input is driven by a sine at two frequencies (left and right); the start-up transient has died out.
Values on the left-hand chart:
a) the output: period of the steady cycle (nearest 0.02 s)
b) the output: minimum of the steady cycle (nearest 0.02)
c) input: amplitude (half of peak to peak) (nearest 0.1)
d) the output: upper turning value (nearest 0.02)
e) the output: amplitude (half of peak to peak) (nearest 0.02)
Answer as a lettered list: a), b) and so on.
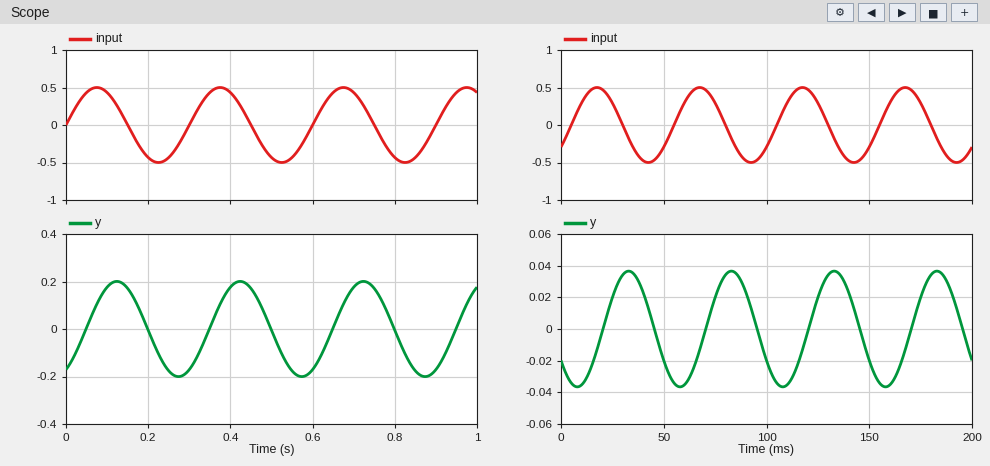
a) 0.30 s
b) -0.20
c) 0.5
d) 0.20
e) 0.20
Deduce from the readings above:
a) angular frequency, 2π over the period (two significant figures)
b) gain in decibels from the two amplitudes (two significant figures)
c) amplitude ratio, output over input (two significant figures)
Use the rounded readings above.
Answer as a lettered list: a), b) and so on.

a) 21 rad/s
b) -8.0 dB
c) 0.40
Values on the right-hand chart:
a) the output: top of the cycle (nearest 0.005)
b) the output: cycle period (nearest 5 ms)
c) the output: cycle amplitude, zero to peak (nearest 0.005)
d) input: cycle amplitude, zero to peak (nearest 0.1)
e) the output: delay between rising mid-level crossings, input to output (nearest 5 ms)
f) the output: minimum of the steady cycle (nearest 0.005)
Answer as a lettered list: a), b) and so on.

a) 0.035
b) 50 ms
c) 0.035
d) 0.5
e) 15 ms
f) -0.035
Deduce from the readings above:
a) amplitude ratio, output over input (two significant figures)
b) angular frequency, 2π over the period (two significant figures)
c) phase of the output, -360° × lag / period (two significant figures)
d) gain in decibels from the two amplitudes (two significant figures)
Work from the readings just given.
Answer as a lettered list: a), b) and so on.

a) 0.070
b) 0.13 rad/ms
c) -110°
d) -23 dB
